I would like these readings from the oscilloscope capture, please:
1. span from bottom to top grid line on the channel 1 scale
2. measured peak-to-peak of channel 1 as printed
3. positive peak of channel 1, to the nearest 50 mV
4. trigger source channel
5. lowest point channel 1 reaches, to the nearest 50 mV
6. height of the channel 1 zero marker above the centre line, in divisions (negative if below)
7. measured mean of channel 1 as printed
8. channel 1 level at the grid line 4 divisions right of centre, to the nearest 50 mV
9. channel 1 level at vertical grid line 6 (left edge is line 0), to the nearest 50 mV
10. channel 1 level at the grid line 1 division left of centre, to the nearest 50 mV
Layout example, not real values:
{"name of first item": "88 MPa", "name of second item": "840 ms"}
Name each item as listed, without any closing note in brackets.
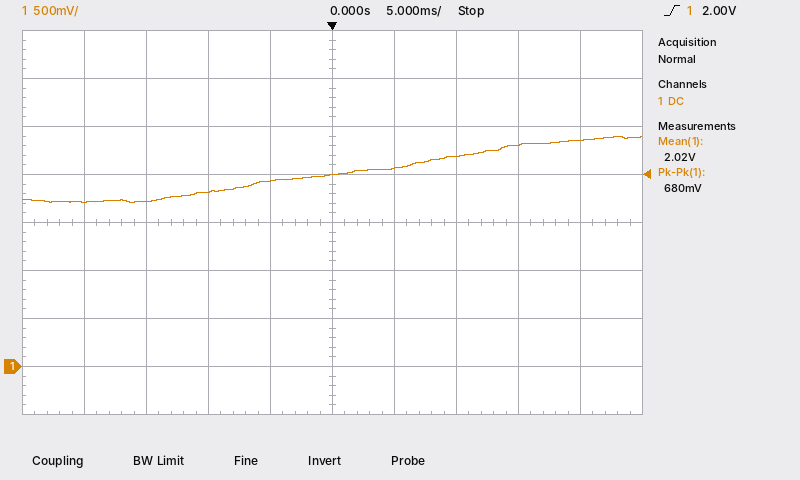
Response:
{"span from bottom to top grid line on the channel 1 scale": "4 V", "measured peak-to-peak of channel 1 as printed": "680 mV", "positive peak of channel 1, to the nearest 50 mV": "2.40 V", "trigger source channel": "channel 1", "lowest point channel 1 reaches, to the nearest 50 mV": "1.70 V", "height of the channel 1 zero marker above the centre line, in divisions": "-3.0 div", "measured mean of channel 1 as printed": "2.02 V", "channel 1 level at the grid line 4 divisions right of centre, to the nearest 50 mV": "2.35 V", "channel 1 level at vertical grid line 6 (left edge is line 0), to the nearest 50 mV": "2.05 V", "channel 1 level at the grid line 1 division left of centre, to the nearest 50 mV": "1.95 V"}
